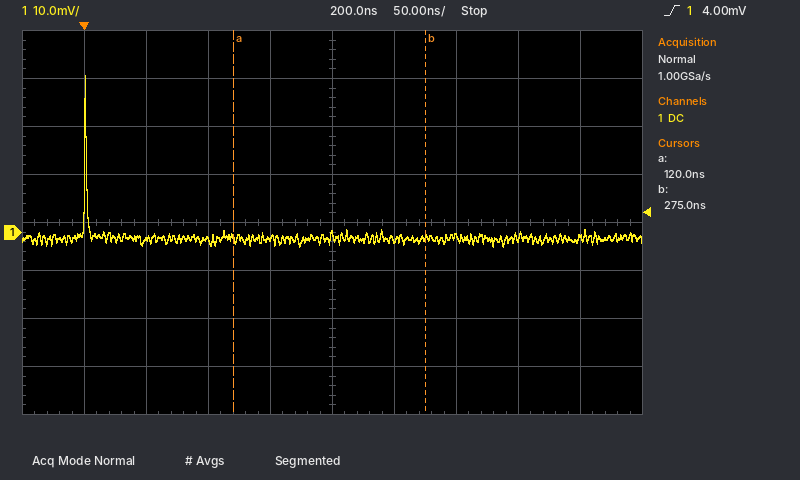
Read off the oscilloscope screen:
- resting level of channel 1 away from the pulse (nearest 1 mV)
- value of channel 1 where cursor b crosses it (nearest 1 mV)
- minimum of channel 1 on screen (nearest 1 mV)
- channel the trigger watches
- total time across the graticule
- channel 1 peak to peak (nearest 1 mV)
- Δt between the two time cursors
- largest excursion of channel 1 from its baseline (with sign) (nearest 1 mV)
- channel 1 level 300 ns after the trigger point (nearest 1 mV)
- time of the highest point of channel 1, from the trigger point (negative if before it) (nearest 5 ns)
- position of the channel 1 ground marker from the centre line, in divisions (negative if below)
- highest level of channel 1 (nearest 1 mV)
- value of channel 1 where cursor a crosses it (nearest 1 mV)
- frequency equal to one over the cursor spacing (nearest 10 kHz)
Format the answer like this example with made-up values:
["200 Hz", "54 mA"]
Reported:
["-1 mV", "-1 mV", "-3 mV", "channel 1", "500 ns", "36 mV", "155 ns", "+34 mV", "-1 mV", "0 ns", "-0.2 div", "33 mV", "-1 mV", "6.45 MHz"]
